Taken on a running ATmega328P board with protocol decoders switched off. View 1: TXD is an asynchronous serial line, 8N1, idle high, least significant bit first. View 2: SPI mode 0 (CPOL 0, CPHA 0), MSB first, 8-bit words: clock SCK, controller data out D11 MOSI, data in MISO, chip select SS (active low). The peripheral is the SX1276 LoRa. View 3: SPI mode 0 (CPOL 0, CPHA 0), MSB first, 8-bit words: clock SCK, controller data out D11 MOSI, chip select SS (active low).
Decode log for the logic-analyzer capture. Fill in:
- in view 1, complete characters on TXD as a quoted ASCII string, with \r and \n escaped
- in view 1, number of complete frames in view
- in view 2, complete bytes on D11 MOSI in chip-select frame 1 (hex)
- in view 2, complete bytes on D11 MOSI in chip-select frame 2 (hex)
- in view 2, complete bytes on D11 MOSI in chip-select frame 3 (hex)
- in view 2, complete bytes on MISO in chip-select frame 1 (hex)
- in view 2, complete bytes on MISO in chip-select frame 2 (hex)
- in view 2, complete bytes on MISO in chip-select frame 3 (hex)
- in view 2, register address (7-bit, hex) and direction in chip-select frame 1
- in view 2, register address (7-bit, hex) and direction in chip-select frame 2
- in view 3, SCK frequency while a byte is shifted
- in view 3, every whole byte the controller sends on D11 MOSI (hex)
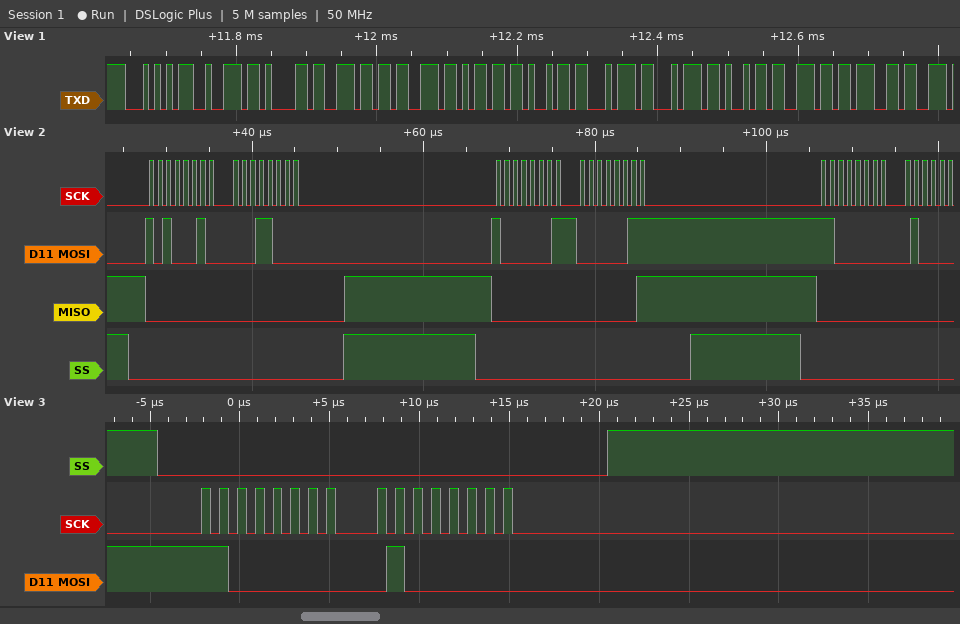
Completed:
"Transmitting"
12
A2 18
81 03
C0
00 00
00 01
00
0x22 write
0x01 write
1 MHz
0xC0 0x40
